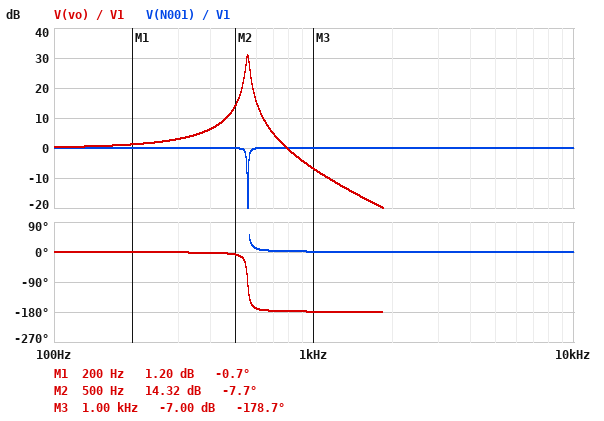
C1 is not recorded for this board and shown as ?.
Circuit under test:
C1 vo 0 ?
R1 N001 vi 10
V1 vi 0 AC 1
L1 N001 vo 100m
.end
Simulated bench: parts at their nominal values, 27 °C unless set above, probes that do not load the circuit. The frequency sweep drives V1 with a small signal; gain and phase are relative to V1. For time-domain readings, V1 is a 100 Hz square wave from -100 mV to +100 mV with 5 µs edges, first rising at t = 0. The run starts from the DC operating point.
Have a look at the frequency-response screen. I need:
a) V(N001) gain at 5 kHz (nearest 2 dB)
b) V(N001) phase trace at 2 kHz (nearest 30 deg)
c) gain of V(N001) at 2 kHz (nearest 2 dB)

0 dB
0 deg
0 dB
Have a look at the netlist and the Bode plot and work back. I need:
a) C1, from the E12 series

820 nF
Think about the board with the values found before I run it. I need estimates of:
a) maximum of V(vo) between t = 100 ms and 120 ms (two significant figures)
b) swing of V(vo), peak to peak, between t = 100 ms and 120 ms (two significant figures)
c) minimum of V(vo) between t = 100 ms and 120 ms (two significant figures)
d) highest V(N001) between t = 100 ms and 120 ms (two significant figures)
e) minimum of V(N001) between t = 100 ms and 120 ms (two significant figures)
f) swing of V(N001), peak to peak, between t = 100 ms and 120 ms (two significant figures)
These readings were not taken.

240 mV
480 mV
-240 mV
100 mV
-100 mV
210 mV
